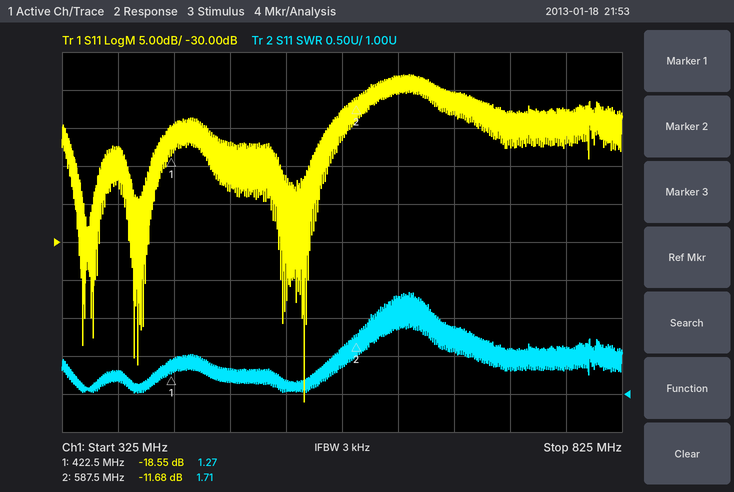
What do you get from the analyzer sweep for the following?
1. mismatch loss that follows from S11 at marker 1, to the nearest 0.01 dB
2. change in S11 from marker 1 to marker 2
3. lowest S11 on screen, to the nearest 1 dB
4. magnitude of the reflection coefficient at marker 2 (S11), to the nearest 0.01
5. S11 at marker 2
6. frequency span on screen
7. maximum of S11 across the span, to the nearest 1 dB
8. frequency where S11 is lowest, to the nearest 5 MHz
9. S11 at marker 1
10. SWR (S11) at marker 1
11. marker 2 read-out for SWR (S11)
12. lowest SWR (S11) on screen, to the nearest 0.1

0.06 dB
6.87 dB
-51 dB
0.26
-11.68 dB
500 MHz
-8 dB
540 MHz
-18.55 dB
1.27
1.71
1.0
